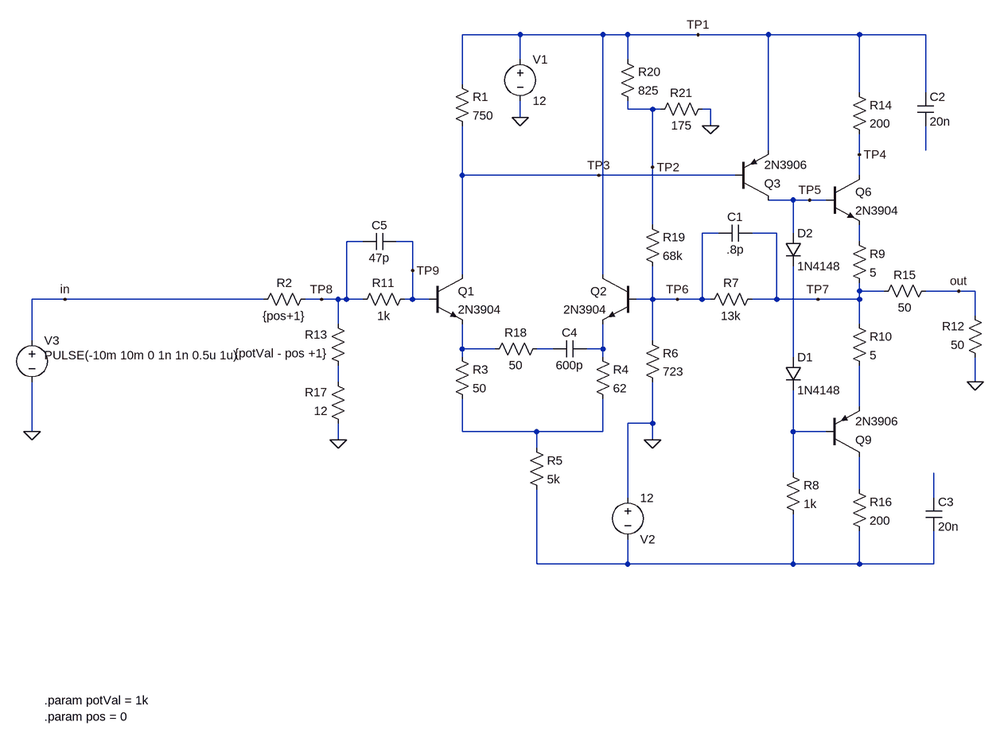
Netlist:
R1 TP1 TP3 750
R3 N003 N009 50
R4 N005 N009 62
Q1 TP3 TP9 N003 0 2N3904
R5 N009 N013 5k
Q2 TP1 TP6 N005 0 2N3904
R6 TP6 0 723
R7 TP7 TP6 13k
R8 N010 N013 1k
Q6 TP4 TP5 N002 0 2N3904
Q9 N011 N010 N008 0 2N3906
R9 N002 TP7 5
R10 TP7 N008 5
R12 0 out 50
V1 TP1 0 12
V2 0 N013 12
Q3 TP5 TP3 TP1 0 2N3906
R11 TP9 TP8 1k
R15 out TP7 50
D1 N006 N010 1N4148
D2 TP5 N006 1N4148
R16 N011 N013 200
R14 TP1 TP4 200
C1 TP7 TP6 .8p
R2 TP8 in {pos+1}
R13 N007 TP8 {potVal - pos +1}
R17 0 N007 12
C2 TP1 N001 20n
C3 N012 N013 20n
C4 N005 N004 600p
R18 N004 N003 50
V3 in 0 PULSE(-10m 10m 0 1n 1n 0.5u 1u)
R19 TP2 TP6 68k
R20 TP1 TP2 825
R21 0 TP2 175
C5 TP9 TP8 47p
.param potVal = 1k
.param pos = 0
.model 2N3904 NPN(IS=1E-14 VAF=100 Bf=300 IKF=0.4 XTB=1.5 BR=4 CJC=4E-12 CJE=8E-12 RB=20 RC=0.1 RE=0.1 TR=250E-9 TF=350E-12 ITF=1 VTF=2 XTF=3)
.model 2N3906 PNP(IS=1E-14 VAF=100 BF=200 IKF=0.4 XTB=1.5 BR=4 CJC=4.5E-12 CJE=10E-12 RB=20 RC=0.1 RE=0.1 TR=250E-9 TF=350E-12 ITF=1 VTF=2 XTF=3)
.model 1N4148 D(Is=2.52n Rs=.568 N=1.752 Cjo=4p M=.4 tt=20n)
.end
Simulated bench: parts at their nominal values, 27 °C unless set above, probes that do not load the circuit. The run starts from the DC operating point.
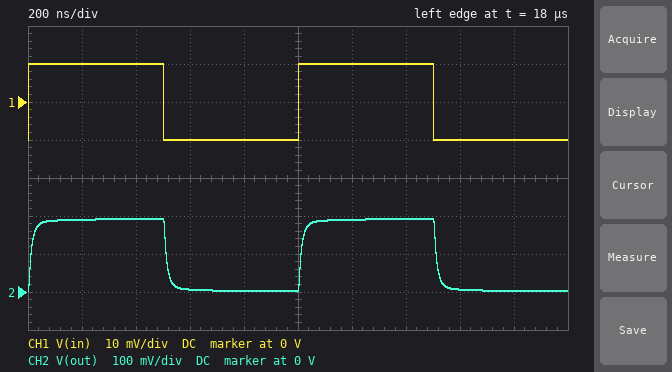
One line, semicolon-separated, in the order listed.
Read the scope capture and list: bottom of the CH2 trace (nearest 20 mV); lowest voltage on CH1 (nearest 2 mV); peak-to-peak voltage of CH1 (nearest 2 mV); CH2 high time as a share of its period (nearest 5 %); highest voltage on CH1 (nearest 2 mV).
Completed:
0 V; -10 mV; 20 mV; 50 %; 10 mV
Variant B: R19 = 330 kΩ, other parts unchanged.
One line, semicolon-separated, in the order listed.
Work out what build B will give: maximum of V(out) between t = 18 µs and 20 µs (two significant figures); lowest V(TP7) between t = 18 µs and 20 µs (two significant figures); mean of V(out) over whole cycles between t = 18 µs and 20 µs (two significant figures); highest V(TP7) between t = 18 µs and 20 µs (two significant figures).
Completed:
340 mV; 310 mV; 250 mV; 690 mV
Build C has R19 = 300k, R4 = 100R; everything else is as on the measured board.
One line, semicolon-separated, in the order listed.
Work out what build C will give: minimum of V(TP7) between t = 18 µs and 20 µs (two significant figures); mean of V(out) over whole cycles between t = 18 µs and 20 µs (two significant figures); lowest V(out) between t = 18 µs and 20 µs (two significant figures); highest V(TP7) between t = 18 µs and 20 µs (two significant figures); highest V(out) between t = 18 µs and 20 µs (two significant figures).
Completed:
1.2 V; 680 mV; 580 mV; 1.5 V; 770 mV
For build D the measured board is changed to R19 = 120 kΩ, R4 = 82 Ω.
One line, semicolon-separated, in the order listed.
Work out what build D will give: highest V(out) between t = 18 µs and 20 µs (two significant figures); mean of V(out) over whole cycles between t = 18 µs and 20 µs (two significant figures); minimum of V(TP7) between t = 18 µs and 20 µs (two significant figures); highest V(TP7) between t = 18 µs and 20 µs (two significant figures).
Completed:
500 mV; 410 mV; 630 mV; 1.0 V
